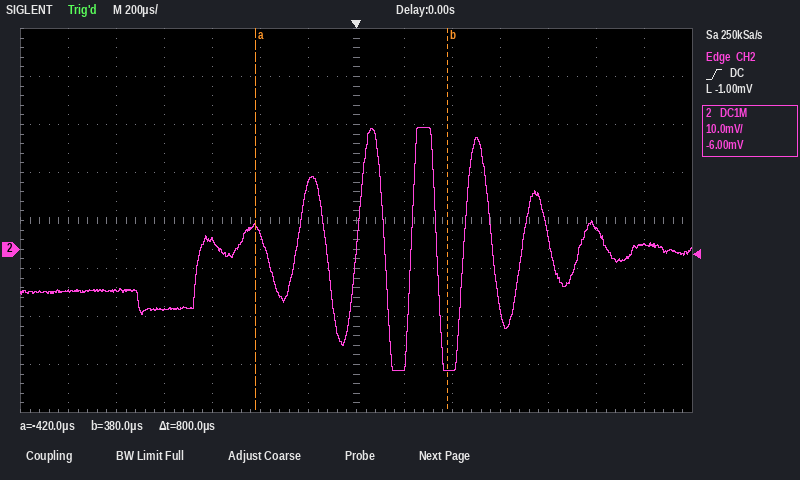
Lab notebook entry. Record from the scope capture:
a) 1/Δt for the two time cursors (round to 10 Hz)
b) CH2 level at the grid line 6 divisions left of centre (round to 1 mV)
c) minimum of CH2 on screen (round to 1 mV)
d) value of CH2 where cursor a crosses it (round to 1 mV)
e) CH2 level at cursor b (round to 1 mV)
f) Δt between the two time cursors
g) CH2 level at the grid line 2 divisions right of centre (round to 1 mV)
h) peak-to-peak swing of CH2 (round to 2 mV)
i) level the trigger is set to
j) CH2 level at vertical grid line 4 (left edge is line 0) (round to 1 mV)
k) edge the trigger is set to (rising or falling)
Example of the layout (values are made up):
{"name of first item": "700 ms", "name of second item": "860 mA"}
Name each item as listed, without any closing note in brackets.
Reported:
{"1/Δt for the two time cursors": "1.25 kHz", "CH2 level at the grid line 6 divisions left of centre": "-9 mV", "minimum of CH2 on screen": "-25 mV", "value of CH2 where cursor a crosses it": "5 mV", "CH2 level at cursor b": "-25 mV", "Δt between the two time cursors": "800 µs", "CH2 level at the grid line 2 divisions right of centre": "-25 mV", "peak-to-peak swing of CH2": "50 mV", "level the trigger is set to": "-1.00 mV", "CH2 level at vertical grid line 4 (left edge is line 0)": "2 mV", "edge the trigger is set to": "rising"}
